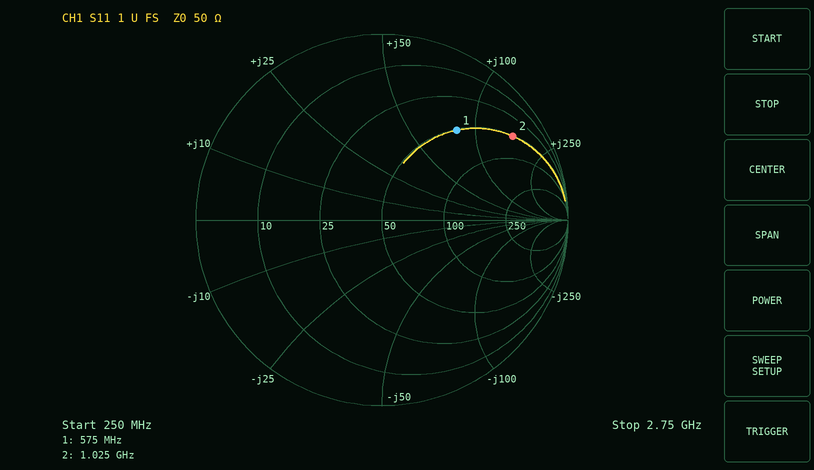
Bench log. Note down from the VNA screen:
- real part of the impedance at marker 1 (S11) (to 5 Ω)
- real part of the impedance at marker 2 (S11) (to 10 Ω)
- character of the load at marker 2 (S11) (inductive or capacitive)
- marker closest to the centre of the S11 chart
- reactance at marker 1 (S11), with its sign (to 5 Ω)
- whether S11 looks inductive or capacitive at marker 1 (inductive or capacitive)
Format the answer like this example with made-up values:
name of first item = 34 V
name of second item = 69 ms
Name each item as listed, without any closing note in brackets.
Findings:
real part of the impedance at marker 1 (S11) = 50 Ω
real part of the impedance at marker 2 (S11) = 50 Ω
character of the load at marker 2 (S11) = inductive
marker closest to the centre of the S11 chart = marker 1
reactance at marker 1 (S11), with its sign = +80 Ω
whether S11 looks inductive or capacitive at marker 1 = inductive
